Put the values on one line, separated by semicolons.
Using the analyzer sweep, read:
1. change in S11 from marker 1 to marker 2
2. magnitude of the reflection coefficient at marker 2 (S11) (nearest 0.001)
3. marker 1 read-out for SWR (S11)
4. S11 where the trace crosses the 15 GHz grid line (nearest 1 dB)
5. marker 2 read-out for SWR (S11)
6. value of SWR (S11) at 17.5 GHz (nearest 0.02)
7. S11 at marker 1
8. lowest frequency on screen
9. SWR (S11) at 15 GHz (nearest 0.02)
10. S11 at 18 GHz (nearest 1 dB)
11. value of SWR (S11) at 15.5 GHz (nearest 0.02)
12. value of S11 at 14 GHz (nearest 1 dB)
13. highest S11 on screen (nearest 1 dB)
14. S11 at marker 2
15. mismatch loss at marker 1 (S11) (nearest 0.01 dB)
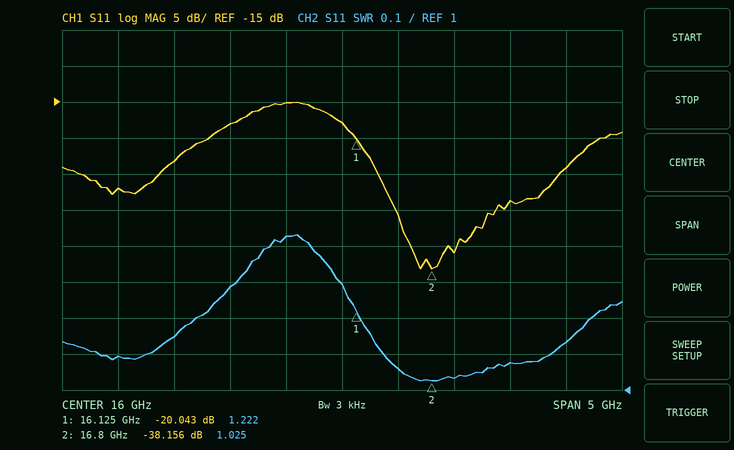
-18.113 dB; 0.012; 1.222; -18 dB; 1.025; 1.08; -20.043 dB; 13.5 GHz; 1.28; -24 dB; 1.42; -27 dB; -15 dB; -38.156 dB; 0.04 dB
